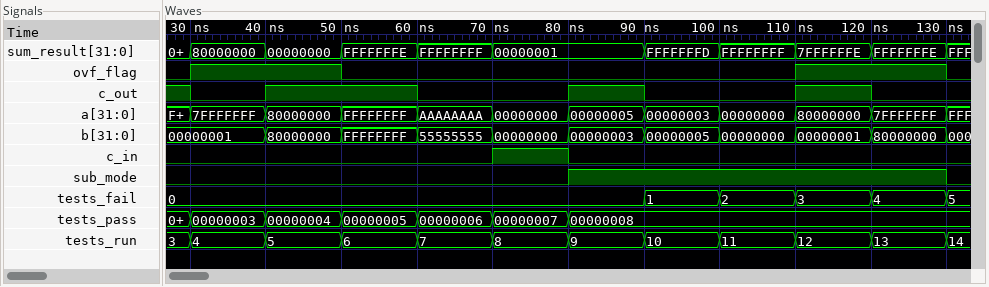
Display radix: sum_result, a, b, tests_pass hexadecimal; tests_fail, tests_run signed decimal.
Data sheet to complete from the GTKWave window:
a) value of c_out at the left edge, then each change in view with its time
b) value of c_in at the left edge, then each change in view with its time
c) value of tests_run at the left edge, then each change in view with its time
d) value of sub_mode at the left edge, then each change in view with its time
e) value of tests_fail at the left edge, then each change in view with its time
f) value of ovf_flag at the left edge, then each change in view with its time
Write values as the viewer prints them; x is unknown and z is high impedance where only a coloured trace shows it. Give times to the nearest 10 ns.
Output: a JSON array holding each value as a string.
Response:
["1, 0 at 30 ns, 1 at 40 ns, 0 at 60 ns, 1 at 80 ns, 0 at 90 ns, 1 at 110 ns, 0 at 120 ns", "0, 1 at 70 ns, 0 at 80 ns", "3, 4 at 30 ns, 5 at 40 ns, 6 at 50 ns, 7 at 60 ns, 8 at 70 ns, 9 at 80 ns, 10 at 90 ns, 11 at 100 ns, 12 at 110 ns, 13 at 120 ns, 14 at 130 ns", "0, 1 at 80 ns, 0 at 130 ns", "0, 1 at 90 ns, 2 at 100 ns, 3 at 110 ns, 4 at 120 ns, 5 at 130 ns", "0, 1 at 30 ns, 0 at 50 ns, 1 at 110 ns, 0 at 130 ns"]
